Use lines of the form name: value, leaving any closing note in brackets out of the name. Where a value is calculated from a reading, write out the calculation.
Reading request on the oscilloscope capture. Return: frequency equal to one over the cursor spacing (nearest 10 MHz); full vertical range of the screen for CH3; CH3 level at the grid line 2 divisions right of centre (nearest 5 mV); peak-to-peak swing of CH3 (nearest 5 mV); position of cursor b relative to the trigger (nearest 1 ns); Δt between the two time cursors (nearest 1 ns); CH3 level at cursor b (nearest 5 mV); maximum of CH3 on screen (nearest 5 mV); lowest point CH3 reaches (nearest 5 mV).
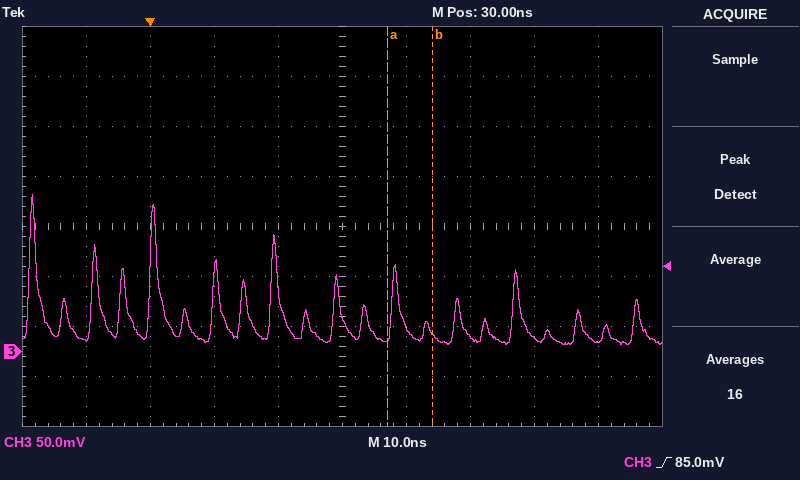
frequency equal to one over the cursor spacing: 1 / 7 ns ≈ 140 MHz
full vertical range of the screen for CH3: 400 mV
CH3 level at the grid line 2 divisions right of centre: 15 mV
peak-to-peak swing of CH3: 155 mV − (5 mV) = 150 mV
position of cursor b relative to the trigger: +44 ns
Δt between the two time cursors: 7 ns
CH3 level at cursor b: 20 mV
maximum of CH3 on screen: 155 mV
lowest point CH3 reaches: 5 mV
